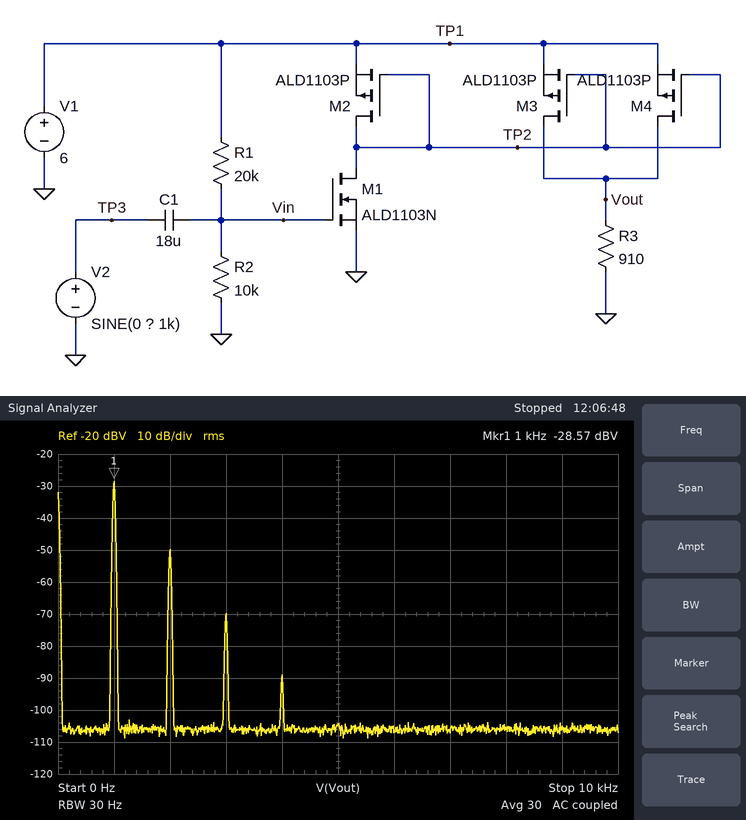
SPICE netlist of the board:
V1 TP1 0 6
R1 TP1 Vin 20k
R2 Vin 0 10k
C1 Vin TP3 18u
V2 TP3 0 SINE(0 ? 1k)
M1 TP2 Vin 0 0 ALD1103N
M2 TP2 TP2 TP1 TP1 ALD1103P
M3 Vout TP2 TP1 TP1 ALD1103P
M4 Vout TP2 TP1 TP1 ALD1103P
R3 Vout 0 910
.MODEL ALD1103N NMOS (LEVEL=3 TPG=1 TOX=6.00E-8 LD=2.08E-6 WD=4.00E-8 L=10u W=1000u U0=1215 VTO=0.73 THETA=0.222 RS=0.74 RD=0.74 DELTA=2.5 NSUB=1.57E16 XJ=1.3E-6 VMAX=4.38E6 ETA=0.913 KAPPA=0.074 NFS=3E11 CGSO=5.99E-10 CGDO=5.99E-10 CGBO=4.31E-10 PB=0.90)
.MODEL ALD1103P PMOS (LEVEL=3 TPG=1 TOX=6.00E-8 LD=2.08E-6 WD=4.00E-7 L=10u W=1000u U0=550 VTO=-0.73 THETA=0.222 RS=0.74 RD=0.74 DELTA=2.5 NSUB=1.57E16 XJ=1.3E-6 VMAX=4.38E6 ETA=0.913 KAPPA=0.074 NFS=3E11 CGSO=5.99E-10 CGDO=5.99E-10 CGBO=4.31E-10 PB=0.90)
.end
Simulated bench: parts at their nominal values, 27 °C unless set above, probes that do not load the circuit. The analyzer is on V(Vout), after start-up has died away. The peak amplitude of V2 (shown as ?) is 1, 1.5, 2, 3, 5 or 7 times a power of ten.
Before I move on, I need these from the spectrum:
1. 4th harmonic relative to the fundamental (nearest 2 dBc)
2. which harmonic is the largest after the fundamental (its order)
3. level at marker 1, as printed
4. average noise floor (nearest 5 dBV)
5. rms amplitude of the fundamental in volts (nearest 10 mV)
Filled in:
-60 dBc
2
-28.57 dBV
-105 dBV
40 mV
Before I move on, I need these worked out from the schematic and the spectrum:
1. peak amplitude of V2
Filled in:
150 mV
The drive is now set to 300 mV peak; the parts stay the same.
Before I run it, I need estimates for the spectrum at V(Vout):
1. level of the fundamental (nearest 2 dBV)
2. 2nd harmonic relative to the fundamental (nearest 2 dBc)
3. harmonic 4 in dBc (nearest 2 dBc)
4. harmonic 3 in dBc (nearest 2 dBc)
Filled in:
-22 dBV
-14 dBc
-40 dBc
-28 dBc
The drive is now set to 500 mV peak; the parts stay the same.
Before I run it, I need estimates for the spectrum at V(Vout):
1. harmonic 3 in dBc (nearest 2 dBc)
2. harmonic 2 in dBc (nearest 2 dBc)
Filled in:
-12 dBc
-6 dBc
